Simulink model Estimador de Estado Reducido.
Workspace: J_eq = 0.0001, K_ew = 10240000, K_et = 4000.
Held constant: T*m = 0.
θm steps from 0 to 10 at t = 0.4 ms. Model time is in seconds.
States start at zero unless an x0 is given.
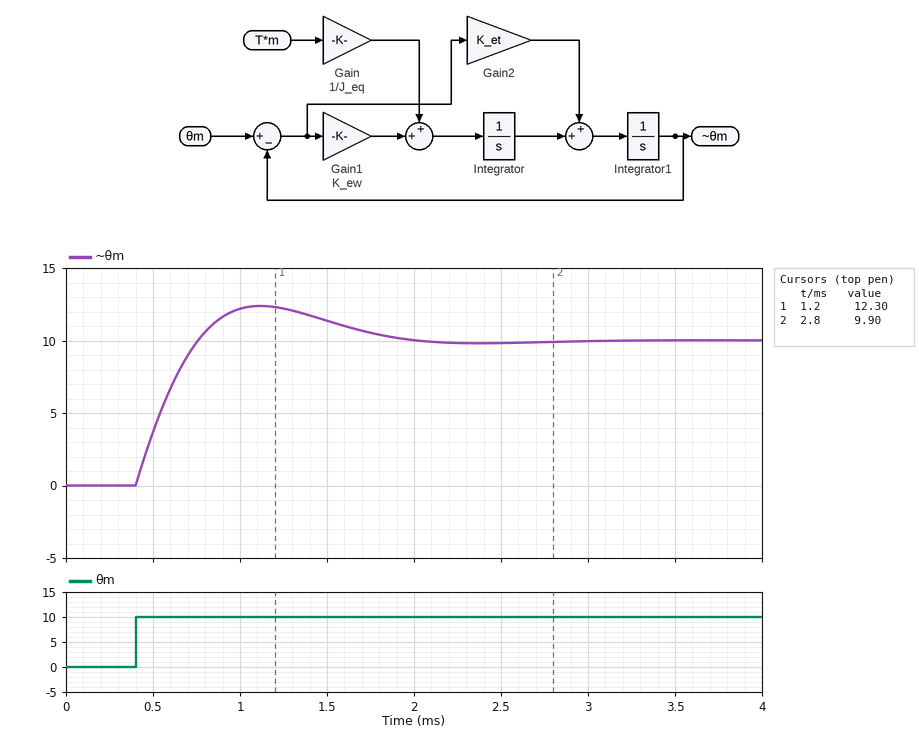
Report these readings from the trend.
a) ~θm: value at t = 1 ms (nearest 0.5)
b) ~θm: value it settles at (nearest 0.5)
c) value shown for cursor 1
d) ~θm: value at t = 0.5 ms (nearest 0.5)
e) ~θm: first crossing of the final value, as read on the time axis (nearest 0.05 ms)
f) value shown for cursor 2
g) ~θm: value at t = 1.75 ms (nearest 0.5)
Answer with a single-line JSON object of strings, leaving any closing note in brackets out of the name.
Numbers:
{"~θm: value at t = 1 ms": "12.0", "~θm: value it settles at": "10.0", "value shown for cursor 1": "12.30", "~θm: value at t = 0.5 ms": "3.5", "~θm: first crossing of the final value, as read on the time axis": "0.75 ms", "value shown for cursor 2": "9.90", "~θm: value at t = 1.75 ms": "10.5"}
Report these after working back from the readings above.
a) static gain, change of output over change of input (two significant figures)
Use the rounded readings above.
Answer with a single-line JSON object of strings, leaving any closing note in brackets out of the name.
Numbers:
{"static gain, change of output over change of input": "1.0"}
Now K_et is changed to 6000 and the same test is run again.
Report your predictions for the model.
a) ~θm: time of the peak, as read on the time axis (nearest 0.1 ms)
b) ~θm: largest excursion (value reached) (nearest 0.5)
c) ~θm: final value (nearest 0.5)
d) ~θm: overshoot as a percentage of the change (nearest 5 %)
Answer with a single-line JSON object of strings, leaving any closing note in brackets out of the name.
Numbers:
{"~θm: time of the peak, as read on the time axis": "1.0 ms", "~θm: largest excursion (value reached)": "11.5", "~θm: final value": "10.0", "~θm: overshoot as a percentage of the change": "15 %"}
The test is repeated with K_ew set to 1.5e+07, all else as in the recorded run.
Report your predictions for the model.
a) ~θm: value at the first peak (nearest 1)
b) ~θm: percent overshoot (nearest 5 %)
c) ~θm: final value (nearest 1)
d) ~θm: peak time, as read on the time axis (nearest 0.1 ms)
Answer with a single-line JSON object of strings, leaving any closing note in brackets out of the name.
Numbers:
{"~θm: value at the first peak": "13", "~θm: percent overshoot": "30 %", "~θm: final value": "10", "~θm: peak time, as read on the time axis": "1.0 ms"}
